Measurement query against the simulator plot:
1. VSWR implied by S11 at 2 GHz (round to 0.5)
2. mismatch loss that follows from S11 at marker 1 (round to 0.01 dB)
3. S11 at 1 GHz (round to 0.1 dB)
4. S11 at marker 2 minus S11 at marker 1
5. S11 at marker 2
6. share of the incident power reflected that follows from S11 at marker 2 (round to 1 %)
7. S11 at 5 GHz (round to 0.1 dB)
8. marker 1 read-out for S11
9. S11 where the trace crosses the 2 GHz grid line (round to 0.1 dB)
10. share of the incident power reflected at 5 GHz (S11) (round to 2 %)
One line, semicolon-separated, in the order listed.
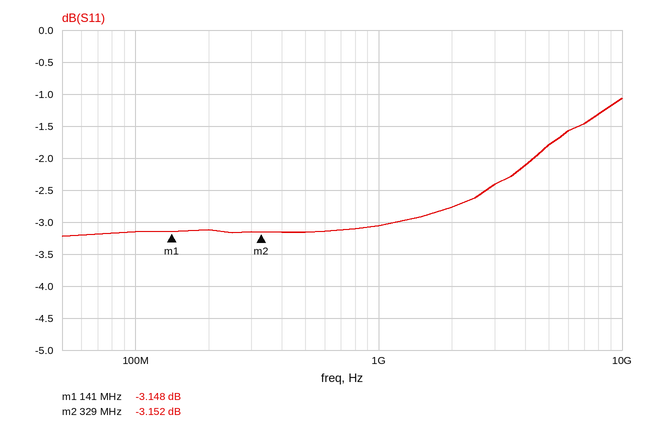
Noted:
6.5; 2.88 dB; -3.1 dB; -0.004 dB; -3.152 dB; 48 %; -1.8 dB; -3.148 dB; -2.8 dB; 66 %
